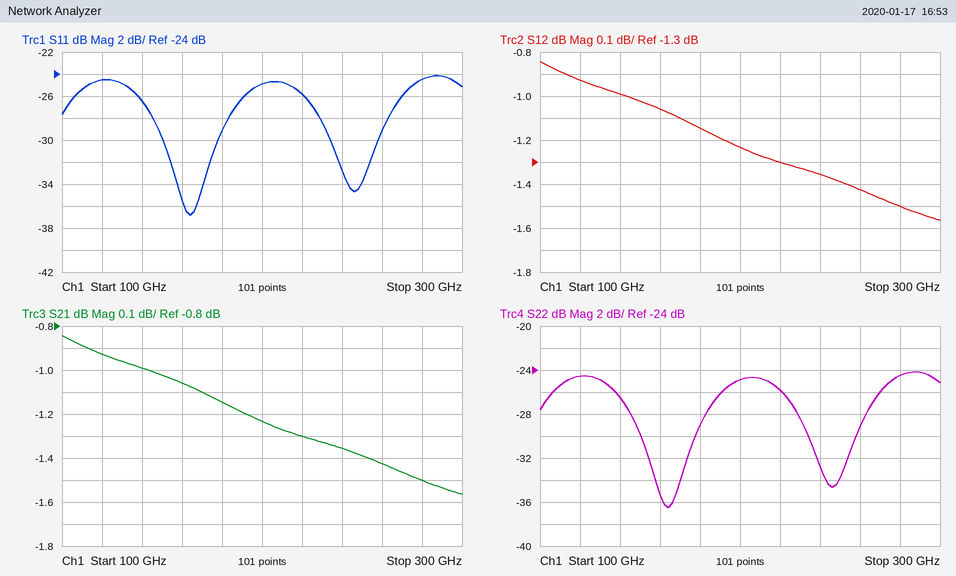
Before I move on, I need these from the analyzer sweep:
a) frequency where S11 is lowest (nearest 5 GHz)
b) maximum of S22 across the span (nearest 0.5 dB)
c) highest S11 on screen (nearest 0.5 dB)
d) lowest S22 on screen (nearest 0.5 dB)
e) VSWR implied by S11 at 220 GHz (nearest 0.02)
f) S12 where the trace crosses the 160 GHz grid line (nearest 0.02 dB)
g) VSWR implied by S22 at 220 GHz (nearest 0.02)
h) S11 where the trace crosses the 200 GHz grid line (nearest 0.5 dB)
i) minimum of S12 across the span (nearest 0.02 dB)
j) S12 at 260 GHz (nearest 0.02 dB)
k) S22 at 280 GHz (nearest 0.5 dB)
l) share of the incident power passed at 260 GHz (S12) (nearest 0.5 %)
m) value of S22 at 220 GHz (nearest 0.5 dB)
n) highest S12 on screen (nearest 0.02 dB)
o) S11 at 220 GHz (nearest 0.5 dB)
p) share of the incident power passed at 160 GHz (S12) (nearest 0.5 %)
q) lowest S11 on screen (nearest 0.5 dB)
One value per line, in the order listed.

165 GHz
-24.0 dB
-24.0 dB
-36.5 dB
1.10
-1.06 dB
1.10
-25.0 dB
-1.56 dB
-1.42 dB
-24.5 dB
72.0 %
-26.0 dB
-0.84 dB
-26.0 dB
78.5 %
-37.0 dB
